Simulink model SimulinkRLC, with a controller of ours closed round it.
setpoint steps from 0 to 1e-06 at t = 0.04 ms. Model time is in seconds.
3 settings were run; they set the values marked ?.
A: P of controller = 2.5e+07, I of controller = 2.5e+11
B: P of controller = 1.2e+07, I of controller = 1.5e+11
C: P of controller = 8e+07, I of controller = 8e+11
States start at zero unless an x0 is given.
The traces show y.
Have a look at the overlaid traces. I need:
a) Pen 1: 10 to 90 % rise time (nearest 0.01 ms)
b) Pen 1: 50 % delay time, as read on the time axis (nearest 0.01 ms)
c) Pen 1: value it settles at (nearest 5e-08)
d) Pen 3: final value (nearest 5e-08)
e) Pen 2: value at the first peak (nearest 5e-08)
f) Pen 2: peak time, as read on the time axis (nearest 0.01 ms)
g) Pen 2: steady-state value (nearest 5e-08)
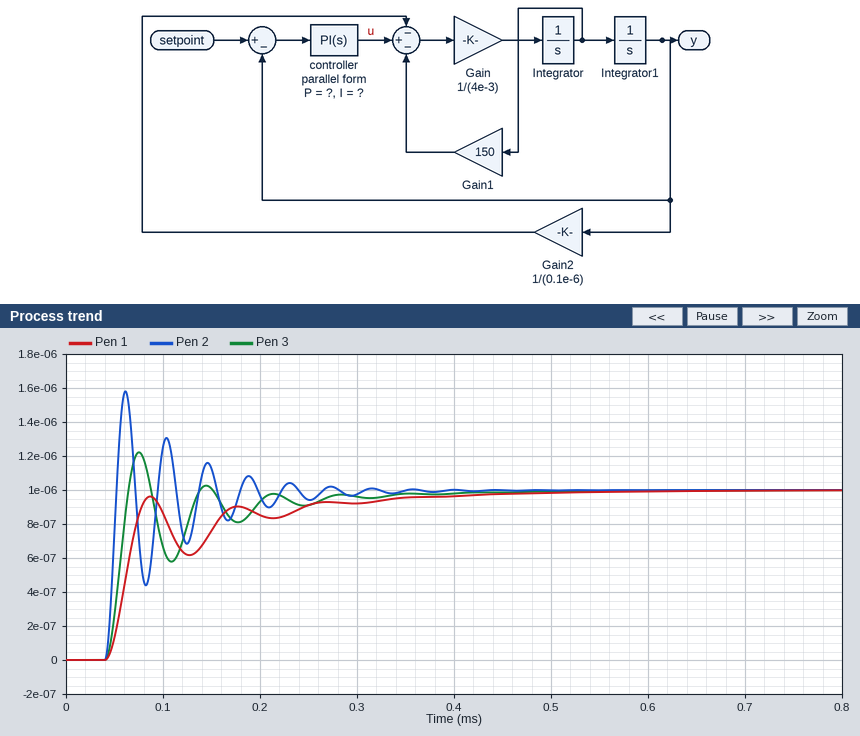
0.03 ms
0.06 ms
0.00000100
0.00000100
0.00000160
0.06 ms
0.00000100
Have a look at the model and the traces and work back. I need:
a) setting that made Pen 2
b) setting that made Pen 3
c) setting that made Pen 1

C
A
B
